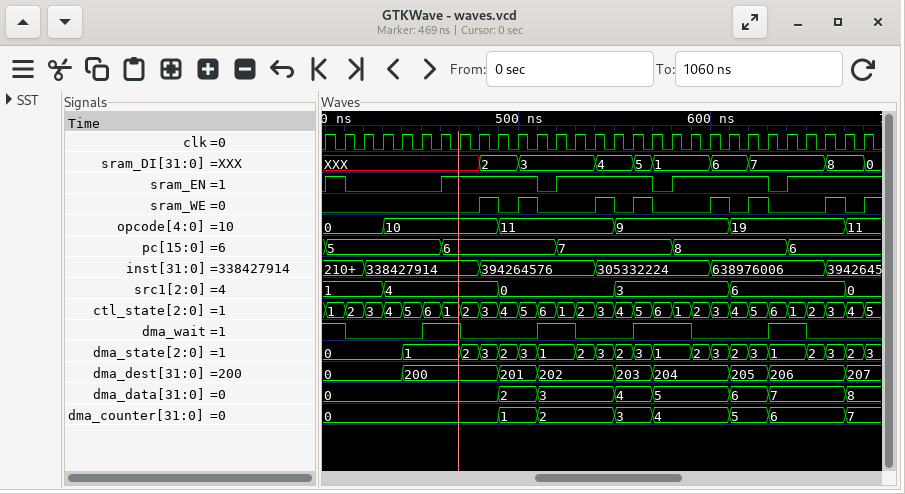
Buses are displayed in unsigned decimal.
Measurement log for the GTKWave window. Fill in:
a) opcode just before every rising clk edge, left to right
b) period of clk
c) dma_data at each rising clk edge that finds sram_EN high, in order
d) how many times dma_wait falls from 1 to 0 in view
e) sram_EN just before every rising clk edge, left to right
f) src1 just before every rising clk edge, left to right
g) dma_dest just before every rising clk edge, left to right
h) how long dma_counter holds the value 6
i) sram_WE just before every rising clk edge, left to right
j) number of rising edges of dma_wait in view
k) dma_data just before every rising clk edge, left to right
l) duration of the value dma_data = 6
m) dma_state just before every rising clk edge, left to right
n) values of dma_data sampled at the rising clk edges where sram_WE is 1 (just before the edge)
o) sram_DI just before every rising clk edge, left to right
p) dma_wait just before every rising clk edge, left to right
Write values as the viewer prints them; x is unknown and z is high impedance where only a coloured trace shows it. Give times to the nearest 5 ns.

0, 0, 0, 0, 10, 10, 10, 10, 10, 10, 11, 11, 11, 11, 11, 11, 9, 9, 9, 9, 9, 9, 19, 19, 19, 19, 19, 19, 11
10 ns
0, 0, 0, 0, 2, 2, 3, 3, 3, 4, 4, 5, 5, 5, 6, 6, 7, 7, 7, 8
5
0 1 0 0 0 0 0 1 1 1 1 1 0 1 1 1 1 1 0 1 1 1 1 1 0 1 1 1 1
1, 1, 1, 1, 4, 4, 4, 4, 4, 4, 0, 0, 0, 0, 0, 0, 3, 3, 3, 3, 3, 3, 6, 6, 6, 6, 6, 6, 0
0, 0, 0, 0, 0, 200, 200, 200, 200, 200, 201, 201, 202, 202, 202, 202, 203, 203, 204, 204, 204, 204, 205, 205, 206, 206, 206, 206, 207
40 ns
0 0 0 0 0 0 0 0 0 1 0 1 0 0 0 1 0 1 0 0 0 1 0 1 0 0 0 1 0
4
0, 0, 0, 0, 0, 0, 0, 0, 0, 0, 2, 2, 3, 3, 3, 3, 4, 4, 5, 5, 5, 5, 6, 6, 7, 7, 7, 7, 8
20 ns
0, 0, 0, 0, 0, 1, 1, 1, 2, 3, 2, 3, 1, 1, 2, 3, 2, 3, 1, 1, 2, 3, 2, 3, 1, 1, 2, 3, 2
0, 2, 3, 4, 5, 6, 7
XXX, XXX, XXX, XXX, XXX, XXX, XXX, XXX, XXX, 2, 2, 3, 3, 3, 3, 4, 4, 5, 1, 1, 1, 6, 6, 7, 7, 7, 7, 8, 8
1 1 0 0 0 0 1 1 0 0 0 0 1 1 0 0 0 1 1 1 0 0 0 0 1 1 0 0 0
